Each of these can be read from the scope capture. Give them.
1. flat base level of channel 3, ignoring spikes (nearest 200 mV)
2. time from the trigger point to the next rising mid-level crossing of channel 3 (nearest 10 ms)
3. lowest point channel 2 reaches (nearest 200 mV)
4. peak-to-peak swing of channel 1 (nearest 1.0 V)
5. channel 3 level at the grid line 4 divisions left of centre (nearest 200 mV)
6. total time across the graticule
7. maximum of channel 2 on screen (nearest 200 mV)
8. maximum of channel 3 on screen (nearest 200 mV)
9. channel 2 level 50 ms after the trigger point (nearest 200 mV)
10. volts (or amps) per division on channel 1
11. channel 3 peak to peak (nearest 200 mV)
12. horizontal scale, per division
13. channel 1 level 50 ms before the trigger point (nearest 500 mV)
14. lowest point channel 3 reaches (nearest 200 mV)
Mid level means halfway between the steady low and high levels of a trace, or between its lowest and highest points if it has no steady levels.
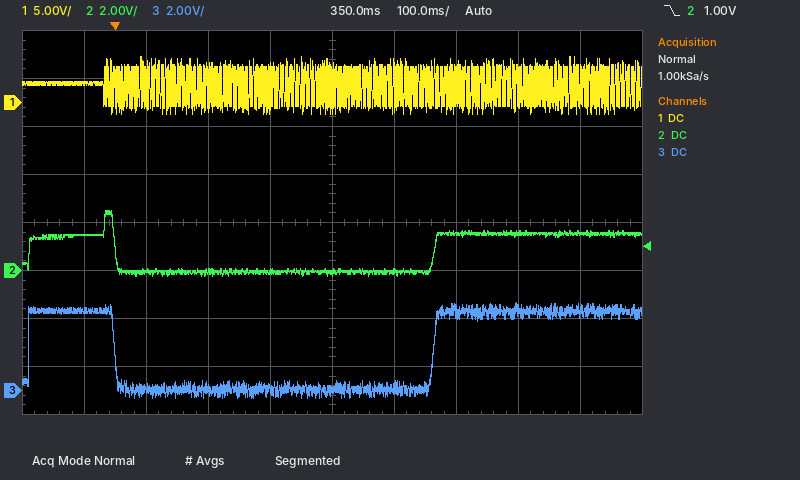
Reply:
0.0 V
510 ms
-200 mV
6.0 V
3.4 V
1 s
2.4 V
3.6 V
0.0 V
5 V
4.0 V
100 ms
2.0 V
-400 mV
